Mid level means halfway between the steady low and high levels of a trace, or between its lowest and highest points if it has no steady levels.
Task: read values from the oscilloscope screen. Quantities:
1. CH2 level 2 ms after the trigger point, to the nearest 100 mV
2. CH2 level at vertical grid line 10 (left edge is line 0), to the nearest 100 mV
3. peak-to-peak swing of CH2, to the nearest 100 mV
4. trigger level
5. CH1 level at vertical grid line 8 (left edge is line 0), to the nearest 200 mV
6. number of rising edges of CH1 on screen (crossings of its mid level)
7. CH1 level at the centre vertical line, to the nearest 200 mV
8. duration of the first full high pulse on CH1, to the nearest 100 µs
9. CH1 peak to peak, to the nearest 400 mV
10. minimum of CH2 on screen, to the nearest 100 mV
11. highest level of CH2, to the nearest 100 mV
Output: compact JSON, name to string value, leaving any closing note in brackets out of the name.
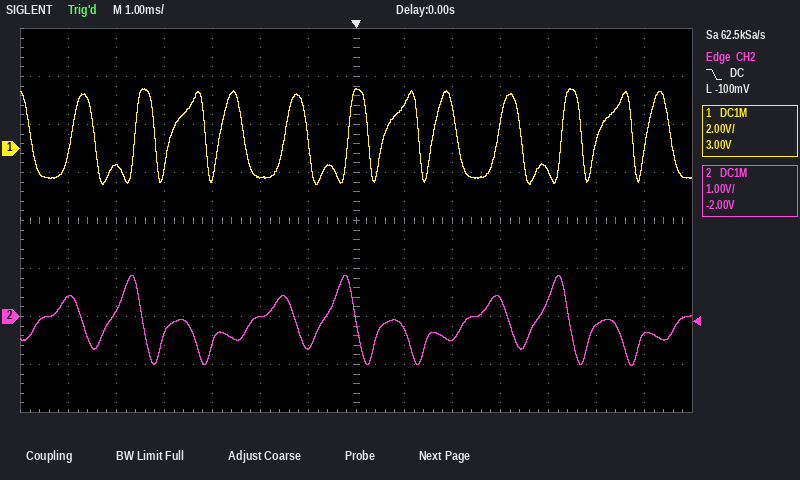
{"CH2 level 2 ms after the trigger point, to the nearest 100 mV": "-500 mV", "CH2 level at vertical grid line 10 (left edge is line 0), to the nearest 100 mV": "400 mV", "peak-to-peak swing of CH2, to the nearest 100 mV": "1.9 V", "trigger level": "-100 mV", "CH1 level at vertical grid line 8 (left edge is line 0), to the nearest 200 mV": "1.8 V", "number of rising edges of CH1 on screen": "12", "CH1 level at the centre vertical line, to the nearest 200 mV": "2.4 V", "duration of the first full high pulse on CH1, to the nearest 100 µs": "500 µs", "CH1 peak to peak, to the nearest 400 mV": "4.0 V", "minimum of CH2 on screen, to the nearest 100 mV": "-1.0 V", "highest level of CH2, to the nearest 100 mV": "900 mV"}
